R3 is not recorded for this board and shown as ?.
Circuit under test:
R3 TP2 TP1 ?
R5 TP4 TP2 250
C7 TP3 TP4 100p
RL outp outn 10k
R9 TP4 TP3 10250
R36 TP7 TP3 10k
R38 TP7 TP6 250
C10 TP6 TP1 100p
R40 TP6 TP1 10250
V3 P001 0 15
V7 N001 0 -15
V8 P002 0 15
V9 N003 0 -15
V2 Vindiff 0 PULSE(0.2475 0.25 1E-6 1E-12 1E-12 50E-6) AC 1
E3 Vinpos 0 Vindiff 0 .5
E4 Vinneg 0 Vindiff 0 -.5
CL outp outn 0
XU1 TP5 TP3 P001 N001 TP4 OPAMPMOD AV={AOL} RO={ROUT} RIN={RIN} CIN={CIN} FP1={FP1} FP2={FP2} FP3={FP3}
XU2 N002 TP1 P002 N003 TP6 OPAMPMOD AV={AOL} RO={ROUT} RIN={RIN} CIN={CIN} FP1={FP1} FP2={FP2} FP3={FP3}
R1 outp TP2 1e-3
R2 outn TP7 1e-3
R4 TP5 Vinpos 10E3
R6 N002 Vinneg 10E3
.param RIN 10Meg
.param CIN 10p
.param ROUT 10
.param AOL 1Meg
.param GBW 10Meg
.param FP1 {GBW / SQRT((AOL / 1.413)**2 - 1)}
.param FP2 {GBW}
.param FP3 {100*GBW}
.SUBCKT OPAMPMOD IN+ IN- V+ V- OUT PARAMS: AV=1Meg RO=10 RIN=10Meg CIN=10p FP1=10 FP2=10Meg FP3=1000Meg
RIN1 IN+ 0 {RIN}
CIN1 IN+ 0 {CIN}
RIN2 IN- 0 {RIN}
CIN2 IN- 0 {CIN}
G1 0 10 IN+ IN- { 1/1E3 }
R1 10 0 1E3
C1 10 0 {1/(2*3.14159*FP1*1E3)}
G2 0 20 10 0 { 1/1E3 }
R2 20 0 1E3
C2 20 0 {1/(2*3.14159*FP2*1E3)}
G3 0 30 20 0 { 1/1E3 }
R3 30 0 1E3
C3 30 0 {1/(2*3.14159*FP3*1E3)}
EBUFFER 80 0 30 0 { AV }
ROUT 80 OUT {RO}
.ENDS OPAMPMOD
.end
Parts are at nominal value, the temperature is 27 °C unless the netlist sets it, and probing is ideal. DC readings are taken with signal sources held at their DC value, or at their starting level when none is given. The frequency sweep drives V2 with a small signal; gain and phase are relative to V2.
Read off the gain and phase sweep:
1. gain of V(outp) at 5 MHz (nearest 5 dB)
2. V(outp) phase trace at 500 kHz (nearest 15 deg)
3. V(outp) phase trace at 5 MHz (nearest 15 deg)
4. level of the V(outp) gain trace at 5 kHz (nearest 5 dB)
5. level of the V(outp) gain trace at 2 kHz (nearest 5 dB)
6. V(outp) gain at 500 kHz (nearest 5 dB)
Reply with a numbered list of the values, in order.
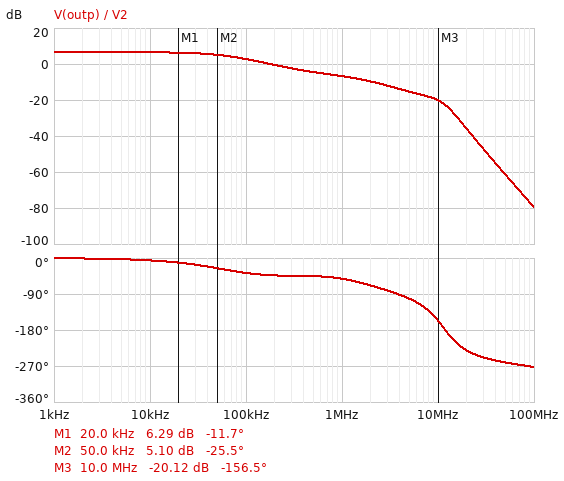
1. -15 dB
2. -45 deg
3. -105 deg
4. 5 dB
5. 5 dB
6. -5 dB
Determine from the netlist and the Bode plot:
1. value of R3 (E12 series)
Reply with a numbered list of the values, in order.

1. 33 kΩ
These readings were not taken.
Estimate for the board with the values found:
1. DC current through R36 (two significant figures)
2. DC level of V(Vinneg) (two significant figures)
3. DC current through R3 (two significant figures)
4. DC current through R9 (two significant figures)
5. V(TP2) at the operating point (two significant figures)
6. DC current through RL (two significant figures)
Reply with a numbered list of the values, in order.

1. 42 µA
2. -120 mV
3. 20 µA
4. 42 µA
5. 530 mV
6. 82 µA
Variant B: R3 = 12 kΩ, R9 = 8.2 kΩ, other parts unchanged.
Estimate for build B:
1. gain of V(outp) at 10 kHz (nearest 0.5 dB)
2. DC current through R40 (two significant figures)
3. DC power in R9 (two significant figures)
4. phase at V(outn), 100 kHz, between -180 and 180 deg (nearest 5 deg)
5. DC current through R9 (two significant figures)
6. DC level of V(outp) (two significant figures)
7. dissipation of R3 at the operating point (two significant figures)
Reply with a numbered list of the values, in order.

1. 11.5 dB
2. 89 µA
3. 96 µW
4. 125 deg
5. 110 µA
6. 940 mV
7. 95 µW
